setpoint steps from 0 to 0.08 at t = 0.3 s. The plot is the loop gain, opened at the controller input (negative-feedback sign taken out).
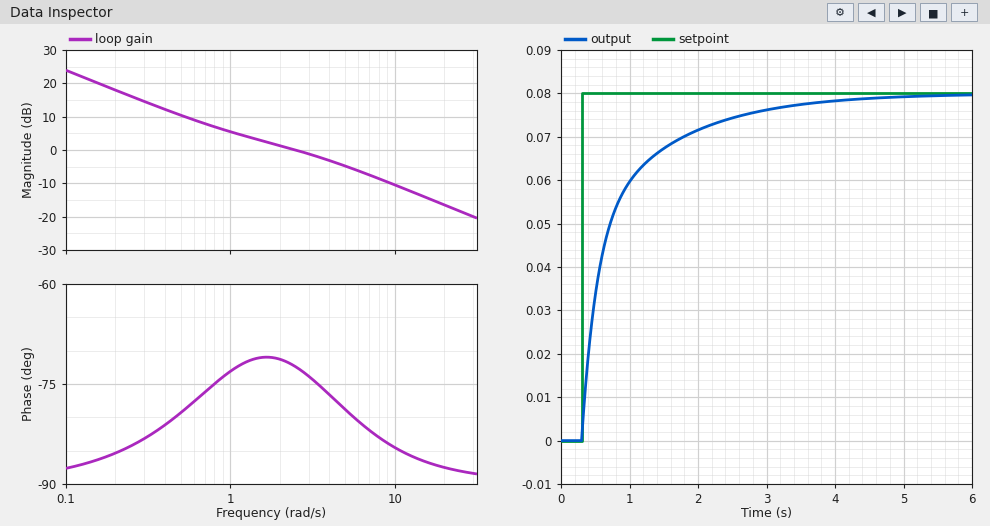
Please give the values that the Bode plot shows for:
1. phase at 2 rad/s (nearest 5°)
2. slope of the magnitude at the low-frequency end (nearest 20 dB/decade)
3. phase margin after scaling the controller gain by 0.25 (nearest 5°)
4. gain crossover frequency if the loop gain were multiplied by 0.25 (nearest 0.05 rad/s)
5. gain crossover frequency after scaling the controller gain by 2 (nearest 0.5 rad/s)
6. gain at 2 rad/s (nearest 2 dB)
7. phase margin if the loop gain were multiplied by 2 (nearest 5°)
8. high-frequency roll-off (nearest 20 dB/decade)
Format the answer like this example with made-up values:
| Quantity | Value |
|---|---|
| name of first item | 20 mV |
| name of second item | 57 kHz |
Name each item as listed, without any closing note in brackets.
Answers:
| Quantity | Value |
|---|---|
| phase at 2 rad/s | -70° |
| slope of the magnitude at the low-frequency end | -20 dB/decade |
| phase margin after scaling the controller gain by 0.25 | 100° |
| gain crossover frequency if the loop gain were multiplied by 0.25 | 0.40 rad/s |
| gain crossover frequency after scaling the controller gain by 2 | 6.0 rad/s |
| gain at 2 rad/s | 2 dB |
| phase margin if the loop gain were multiplied by 2 | 100° |
| high-frequency roll-off | -20 dB/decade |
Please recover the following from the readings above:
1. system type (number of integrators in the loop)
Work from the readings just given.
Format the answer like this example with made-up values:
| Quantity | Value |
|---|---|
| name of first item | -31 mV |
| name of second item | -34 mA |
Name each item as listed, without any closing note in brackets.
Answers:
| Quantity | Value |
|---|---|
| system type | 1 |
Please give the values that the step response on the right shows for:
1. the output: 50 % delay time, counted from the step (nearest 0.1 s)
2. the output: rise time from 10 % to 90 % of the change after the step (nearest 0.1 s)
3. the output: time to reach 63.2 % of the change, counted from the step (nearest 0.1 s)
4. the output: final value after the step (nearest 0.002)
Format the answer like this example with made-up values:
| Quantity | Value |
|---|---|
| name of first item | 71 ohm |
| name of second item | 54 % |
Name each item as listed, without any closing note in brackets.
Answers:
| Quantity | Value |
|---|---|
| the output: 50 % delay time, counted from the step | 0.3 s |
| the output: rise time from 10 % to 90 % of the change after the step | 1.7 s |
| the output: time to reach 63.2 % of the change, counted from the step | 0.4 s |
| the output: final value after the step | 0.080 |
